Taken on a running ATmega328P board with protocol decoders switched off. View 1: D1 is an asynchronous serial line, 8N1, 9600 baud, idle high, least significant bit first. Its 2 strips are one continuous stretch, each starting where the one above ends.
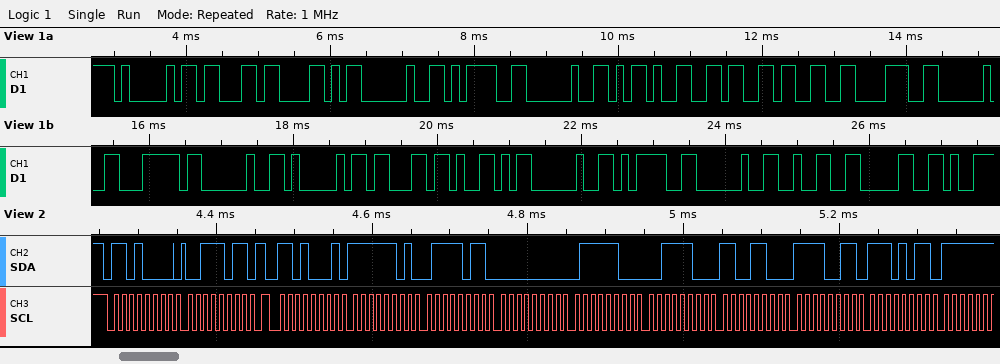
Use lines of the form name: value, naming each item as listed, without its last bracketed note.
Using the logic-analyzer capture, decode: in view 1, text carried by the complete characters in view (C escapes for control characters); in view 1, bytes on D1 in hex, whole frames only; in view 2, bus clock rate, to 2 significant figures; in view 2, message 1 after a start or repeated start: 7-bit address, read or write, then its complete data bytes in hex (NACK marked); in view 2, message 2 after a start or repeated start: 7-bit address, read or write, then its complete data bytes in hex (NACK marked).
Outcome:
in view 1, text carried by the complete characters in view: "AcX = -638 | AcY = 20"
in view 1, bytes on D1 in hex, whole frames only: 41 63 58 20 3D 20 2D 36 33 38 20 7C 20 41 63 59 20 3D 20 32 30
in view 2, bus clock rate, to 2 significant figures: 100 kHz
in view 2, message 1 after a start or repeated start: 7-bit address, read or write, then its complete data bytes in hex: 0x68 write: 3B
in view 2, message 2 after a start or repeated start: 7-bit address, read or write, then its complete data bytes in hex: 0x68 read: FD 7B 00 7C 3C CC F3 EB
